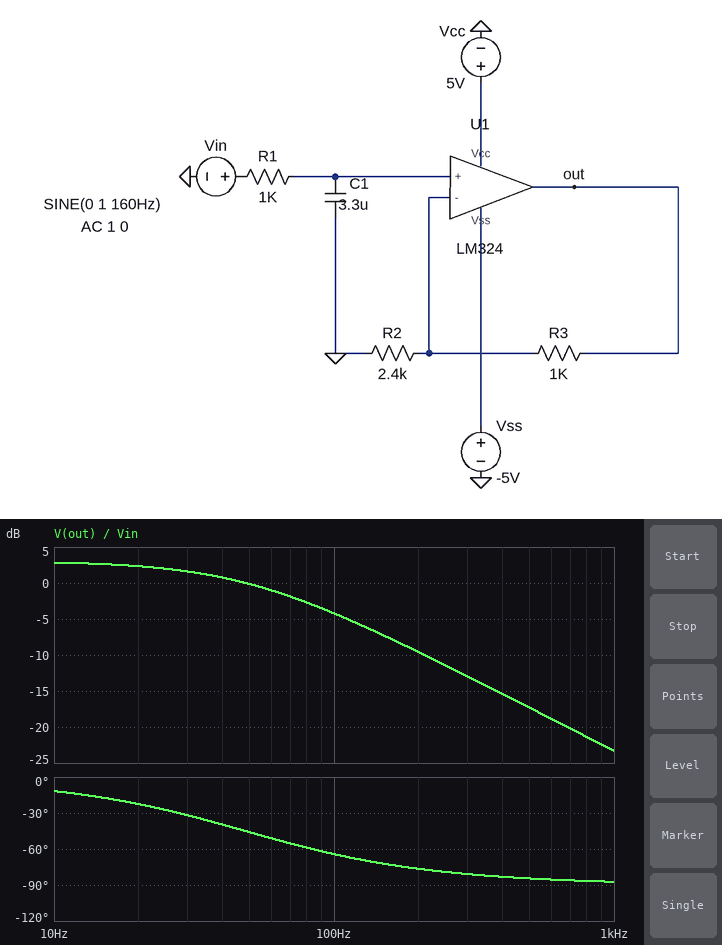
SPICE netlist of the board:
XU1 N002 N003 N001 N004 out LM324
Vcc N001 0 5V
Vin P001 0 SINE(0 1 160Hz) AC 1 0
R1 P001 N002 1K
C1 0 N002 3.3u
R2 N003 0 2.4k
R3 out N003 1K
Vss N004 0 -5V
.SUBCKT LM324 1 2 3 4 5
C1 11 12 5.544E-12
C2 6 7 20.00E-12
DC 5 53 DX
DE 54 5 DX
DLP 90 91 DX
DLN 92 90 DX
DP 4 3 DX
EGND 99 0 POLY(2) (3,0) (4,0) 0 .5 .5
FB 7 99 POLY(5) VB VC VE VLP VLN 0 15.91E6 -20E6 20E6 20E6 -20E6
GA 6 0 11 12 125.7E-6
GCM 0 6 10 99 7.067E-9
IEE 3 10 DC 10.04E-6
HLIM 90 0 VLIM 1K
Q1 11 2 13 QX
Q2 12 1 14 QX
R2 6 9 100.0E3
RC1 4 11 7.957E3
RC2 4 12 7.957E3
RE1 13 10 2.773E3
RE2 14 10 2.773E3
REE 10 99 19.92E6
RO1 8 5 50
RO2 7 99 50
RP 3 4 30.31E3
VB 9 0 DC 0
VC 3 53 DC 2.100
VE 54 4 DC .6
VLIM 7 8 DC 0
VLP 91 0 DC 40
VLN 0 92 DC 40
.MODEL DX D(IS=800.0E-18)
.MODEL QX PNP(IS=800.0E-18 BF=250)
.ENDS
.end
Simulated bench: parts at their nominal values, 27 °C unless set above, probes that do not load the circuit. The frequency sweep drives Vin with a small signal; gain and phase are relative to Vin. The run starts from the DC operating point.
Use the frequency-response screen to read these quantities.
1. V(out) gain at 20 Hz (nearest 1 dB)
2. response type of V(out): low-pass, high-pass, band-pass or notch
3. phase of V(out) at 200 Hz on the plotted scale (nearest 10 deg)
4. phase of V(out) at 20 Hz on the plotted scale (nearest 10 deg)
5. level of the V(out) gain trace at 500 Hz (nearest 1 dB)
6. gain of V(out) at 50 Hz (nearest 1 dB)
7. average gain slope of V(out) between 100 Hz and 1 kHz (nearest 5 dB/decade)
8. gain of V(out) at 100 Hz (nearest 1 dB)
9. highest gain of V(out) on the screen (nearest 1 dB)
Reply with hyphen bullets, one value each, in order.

- 2 dB
- low-pass
- -80 deg
- -20 deg
- -17 dB
- 0 dB
- -20 dB/decade
- -4 dB
- 3 dB
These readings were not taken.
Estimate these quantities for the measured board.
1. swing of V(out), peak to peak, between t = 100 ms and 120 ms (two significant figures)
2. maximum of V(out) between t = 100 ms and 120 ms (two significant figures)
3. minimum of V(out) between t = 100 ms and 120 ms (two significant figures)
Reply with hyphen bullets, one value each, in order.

- 820 mV
- 410 mV
- -410 mV
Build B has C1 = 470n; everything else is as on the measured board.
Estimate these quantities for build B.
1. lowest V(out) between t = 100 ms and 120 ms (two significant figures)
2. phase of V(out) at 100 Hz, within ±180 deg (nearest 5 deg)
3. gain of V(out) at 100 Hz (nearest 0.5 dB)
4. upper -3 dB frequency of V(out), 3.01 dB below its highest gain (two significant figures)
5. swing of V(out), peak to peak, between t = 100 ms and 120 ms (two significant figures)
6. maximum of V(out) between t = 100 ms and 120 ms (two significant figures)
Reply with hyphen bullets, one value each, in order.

- -1.3 V
- -15 deg
- 2.5 dB
- 340 Hz
- 2.6 V
- 1.3 V
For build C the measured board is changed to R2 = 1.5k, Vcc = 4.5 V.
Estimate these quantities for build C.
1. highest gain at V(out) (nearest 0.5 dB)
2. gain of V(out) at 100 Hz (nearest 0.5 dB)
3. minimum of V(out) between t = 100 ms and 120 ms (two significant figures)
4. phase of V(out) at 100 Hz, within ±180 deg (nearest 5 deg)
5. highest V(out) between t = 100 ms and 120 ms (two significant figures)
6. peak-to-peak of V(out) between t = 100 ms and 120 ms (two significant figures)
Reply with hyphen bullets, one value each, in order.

- 4.5 dB
- -3.0 dB
- -480 mV
- -65 deg
- 480 mV
- 960 mV
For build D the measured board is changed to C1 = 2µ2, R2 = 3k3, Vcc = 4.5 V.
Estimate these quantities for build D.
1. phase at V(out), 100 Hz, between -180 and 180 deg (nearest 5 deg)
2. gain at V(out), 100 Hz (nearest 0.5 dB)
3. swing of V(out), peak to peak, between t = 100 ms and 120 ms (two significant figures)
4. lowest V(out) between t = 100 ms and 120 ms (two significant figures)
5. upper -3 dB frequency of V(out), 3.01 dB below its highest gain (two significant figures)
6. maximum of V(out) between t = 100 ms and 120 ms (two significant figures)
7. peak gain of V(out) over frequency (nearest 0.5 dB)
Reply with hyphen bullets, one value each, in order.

- -55 deg
- -2.5 dB
- 1.1 V
- -540 mV
- 72 Hz
- 540 mV
- 2.5 dB
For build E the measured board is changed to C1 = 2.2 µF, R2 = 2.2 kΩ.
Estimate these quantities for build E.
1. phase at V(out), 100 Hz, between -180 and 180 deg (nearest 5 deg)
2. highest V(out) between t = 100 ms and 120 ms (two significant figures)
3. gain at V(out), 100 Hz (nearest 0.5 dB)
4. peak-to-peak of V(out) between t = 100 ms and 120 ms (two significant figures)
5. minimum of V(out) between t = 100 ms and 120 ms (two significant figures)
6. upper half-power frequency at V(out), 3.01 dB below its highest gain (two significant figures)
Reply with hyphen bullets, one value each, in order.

- -55 deg
- 600 mV
- -1.5 dB
- 1.2 V
- -600 mV
- 72 Hz
